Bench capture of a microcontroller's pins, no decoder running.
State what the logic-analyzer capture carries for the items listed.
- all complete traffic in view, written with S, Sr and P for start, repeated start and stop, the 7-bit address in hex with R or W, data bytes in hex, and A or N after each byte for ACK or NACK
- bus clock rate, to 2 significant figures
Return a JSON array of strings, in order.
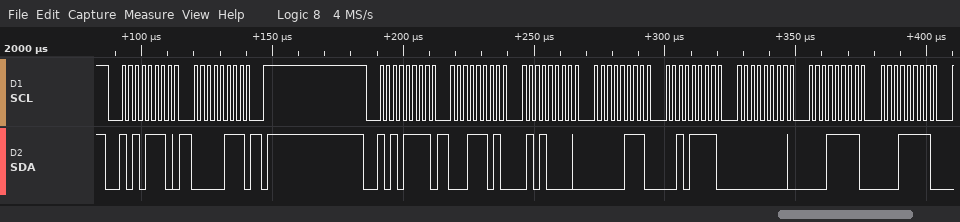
["S 57W A 07 A P S 57R A 1D A 50 A 07 A 2F A 00 A 1F A 1F A", "400 kHz"]
